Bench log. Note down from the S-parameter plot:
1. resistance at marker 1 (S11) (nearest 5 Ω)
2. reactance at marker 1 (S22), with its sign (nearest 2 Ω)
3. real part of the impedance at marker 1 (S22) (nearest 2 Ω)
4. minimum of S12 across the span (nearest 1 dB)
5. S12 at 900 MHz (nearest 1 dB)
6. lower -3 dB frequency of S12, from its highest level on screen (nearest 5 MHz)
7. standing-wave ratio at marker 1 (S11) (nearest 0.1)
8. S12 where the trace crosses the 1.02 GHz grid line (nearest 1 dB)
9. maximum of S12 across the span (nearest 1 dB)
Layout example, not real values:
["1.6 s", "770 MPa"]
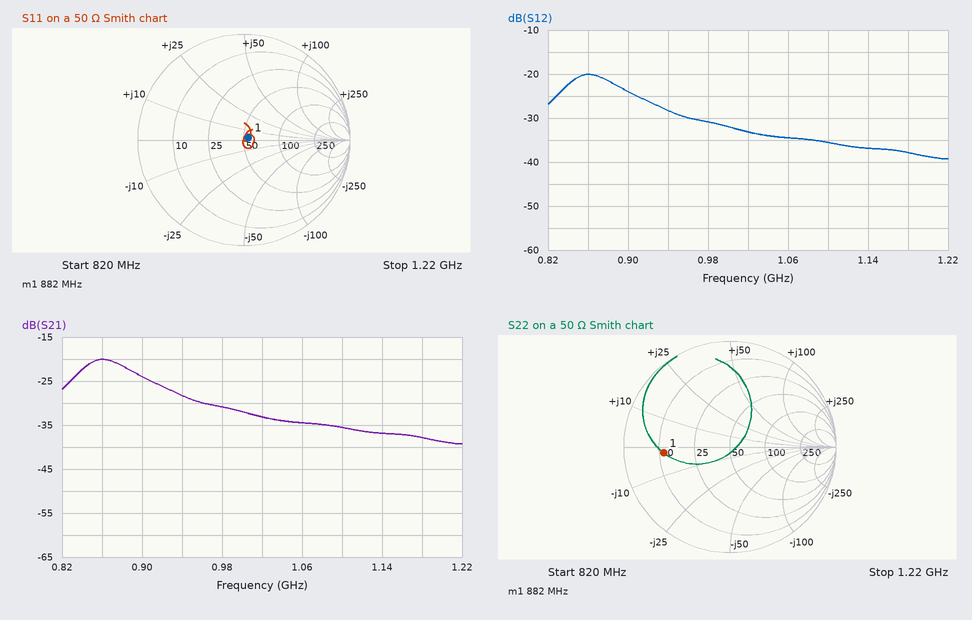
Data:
["55 Ω", "-2 Ω", "12 Ω", "-39 dB", "-24 dB", "835 MHz", "1.1", "-33 dB", "-20 dB"]
